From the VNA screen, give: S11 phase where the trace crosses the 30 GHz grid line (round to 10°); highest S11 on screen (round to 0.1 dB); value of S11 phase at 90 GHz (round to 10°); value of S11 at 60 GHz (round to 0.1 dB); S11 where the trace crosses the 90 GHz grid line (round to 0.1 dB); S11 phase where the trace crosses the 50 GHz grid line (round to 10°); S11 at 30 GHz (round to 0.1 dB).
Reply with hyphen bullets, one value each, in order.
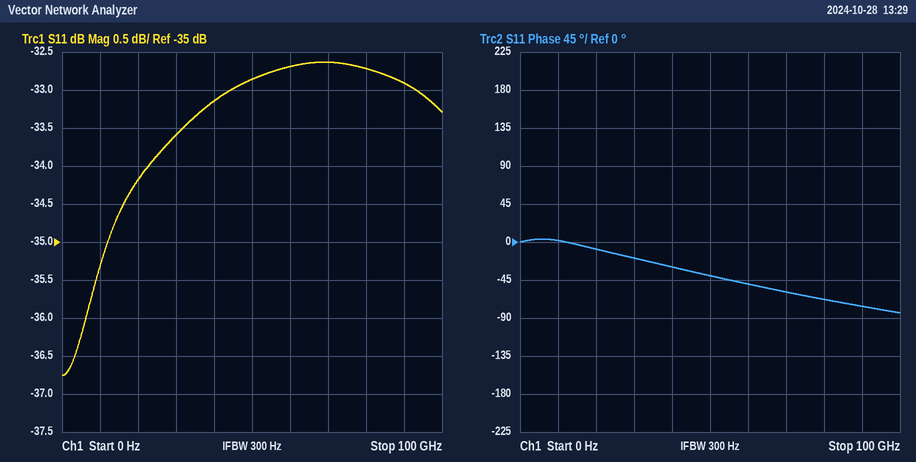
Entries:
- -20°
- -32.6 dB
- -80°
- -32.7 dB
- -32.9 dB
- -40°
- -33.6 dB
